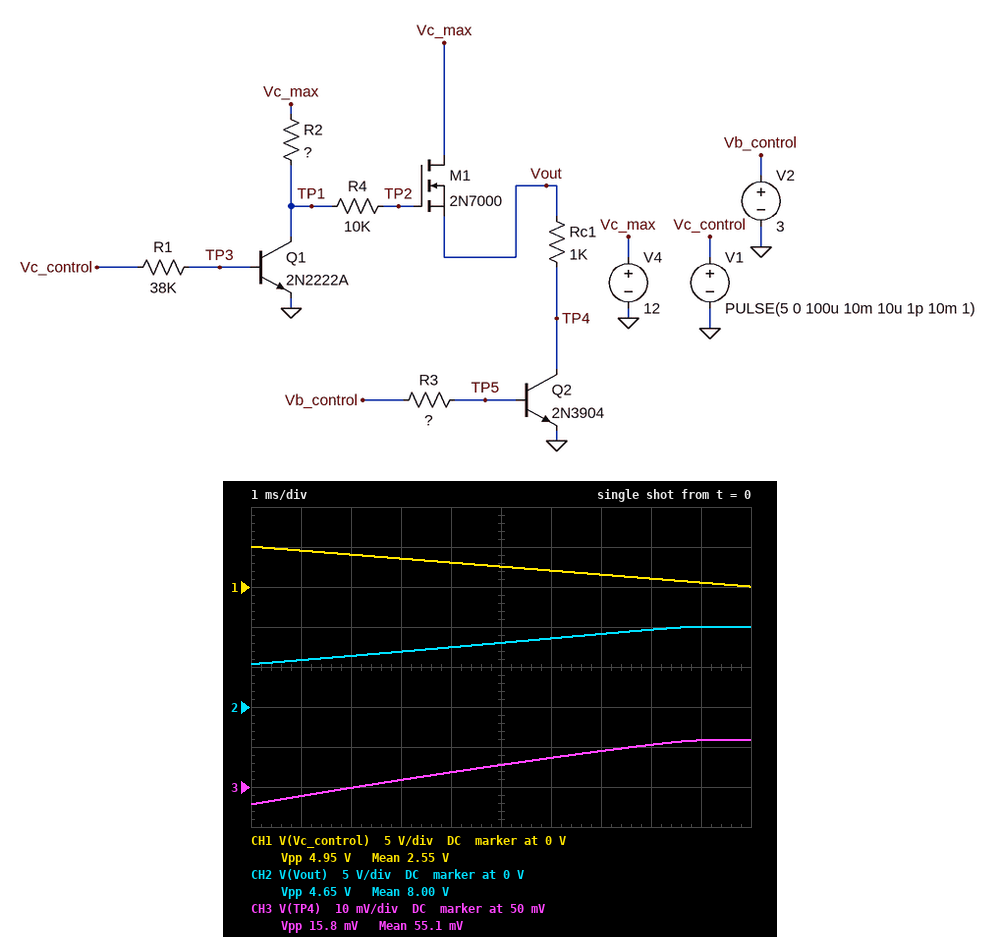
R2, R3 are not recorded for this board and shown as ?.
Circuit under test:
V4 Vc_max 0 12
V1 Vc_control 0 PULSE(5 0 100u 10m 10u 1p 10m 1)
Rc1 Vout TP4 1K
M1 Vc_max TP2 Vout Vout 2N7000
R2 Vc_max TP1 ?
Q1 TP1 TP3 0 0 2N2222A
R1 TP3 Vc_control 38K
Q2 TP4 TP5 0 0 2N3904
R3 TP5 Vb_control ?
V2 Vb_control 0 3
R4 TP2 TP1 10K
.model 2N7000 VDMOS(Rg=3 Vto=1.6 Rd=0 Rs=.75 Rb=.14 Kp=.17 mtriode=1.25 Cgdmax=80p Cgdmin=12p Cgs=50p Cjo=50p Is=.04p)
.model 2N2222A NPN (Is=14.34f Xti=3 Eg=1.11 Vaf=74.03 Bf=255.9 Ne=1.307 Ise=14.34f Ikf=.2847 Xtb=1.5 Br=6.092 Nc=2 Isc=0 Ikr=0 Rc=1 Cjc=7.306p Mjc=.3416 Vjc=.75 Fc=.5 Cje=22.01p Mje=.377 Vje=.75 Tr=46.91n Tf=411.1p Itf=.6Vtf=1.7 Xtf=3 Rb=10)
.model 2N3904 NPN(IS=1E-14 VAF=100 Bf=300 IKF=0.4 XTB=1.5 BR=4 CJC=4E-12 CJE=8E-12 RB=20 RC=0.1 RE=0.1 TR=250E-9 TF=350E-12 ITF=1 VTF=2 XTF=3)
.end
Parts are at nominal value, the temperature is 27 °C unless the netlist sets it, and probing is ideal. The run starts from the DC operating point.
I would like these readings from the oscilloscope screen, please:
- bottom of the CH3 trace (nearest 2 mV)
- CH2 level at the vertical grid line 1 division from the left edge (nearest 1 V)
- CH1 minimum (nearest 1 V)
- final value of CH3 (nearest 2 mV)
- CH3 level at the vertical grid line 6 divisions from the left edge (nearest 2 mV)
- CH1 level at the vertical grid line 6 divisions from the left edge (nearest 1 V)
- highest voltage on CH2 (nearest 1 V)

46 mV
6 V
0 V
62 mV
58 mV
2 V
10 V
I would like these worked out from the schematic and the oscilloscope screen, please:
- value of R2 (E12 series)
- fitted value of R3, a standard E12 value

220 Ω
6.8 kΩ
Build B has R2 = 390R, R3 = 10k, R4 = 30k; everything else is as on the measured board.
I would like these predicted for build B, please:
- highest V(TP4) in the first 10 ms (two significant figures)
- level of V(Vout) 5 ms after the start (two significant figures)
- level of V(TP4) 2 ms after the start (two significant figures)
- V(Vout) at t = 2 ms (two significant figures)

72 mV
6.5 V
46 mV
3.8 V
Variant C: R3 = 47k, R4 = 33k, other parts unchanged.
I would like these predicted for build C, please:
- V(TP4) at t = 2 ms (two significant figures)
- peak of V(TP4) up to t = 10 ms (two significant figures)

110 mV
140 mV
